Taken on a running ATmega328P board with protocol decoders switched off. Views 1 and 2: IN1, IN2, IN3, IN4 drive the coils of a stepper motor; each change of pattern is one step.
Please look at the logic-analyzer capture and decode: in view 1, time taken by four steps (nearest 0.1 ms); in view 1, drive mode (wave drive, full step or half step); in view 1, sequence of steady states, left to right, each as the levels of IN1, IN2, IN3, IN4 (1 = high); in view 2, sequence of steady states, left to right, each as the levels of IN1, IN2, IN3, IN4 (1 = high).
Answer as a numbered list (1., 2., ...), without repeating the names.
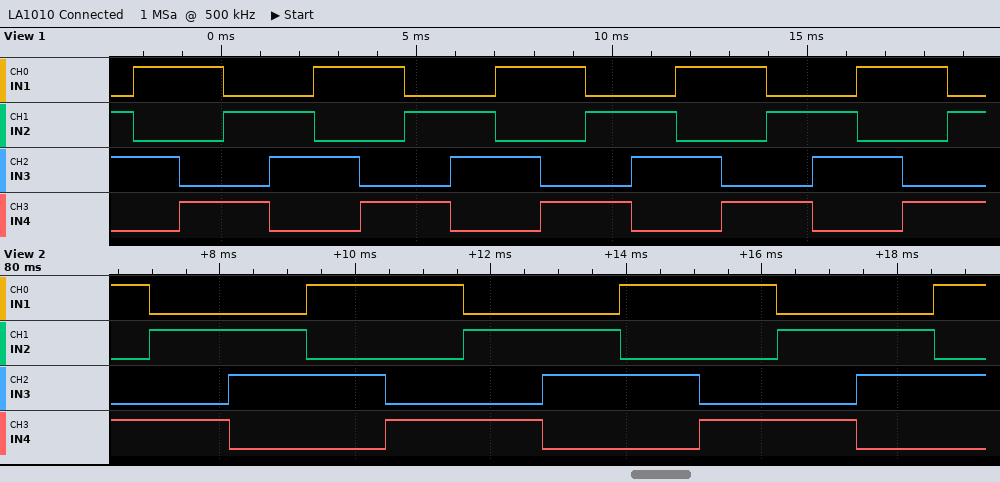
1. 4.6 ms
2. full step
3. 0110 1010 1001 0101 0110 1010 1001 0101 0110 1010 1001 0101 0110 1010 1001 0101 0110 1010 1001 0101
4. 1001 0101 0110 1010 1001 0101 0110 1010 1001 0101 0110 1010
